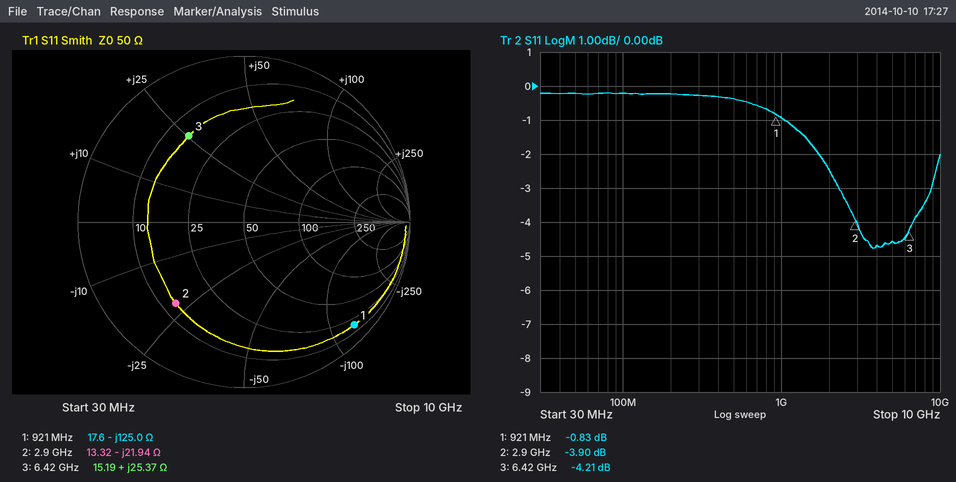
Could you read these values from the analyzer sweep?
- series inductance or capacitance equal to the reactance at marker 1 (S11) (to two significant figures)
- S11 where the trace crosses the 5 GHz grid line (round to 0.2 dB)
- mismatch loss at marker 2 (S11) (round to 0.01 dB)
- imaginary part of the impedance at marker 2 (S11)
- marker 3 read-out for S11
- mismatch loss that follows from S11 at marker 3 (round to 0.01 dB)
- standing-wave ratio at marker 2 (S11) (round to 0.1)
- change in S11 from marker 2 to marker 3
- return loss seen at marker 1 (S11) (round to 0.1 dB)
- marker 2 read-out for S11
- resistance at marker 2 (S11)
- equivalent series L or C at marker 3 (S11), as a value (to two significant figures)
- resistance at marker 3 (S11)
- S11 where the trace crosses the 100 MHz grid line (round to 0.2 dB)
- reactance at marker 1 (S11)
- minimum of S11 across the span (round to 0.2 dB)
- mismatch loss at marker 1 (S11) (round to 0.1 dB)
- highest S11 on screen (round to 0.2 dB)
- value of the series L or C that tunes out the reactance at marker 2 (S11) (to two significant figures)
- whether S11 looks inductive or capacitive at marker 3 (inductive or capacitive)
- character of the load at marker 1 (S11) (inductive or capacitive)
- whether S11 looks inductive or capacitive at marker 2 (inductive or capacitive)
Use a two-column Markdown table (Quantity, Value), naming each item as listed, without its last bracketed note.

| Quantity | Value |
|---|---|
| series inductance or capacitance equal to the reactance at marker 1 (S11) | 1.4 pF |
| S11 where the trace crosses the 5 GHz grid line | -4.6 dB |
| mismatch loss at marker 2 (S11) | 2.27 dB |
| imaginary part of the impedance at marker 2 | -21.94 Ω |
| marker 3 read-out for S11 | -4.21 dB |
| mismatch loss that follows from S11 at marker 3 | 2.07 dB |
| standing-wave ratio at marker 2 (S11) | 4.5 |
| change in S11 from marker 2 to marker 3 | -0.31 dB |
| return loss seen at marker 1 (S11) | 0.8 dB |
| marker 2 read-out for S11 | -3.90 dB |
| resistance at marker 2 | 13.32 Ω |
| equivalent series L or C at marker 3 (S11), as a value | 630 pH |
| resistance at marker 3 | 15.19 Ω |
| S11 where the trace crosses the 100 MHz grid line | -0.2 dB |
| reactance at marker 1 | -125.0 Ω |
| minimum of S11 across the span | -4.8 dB |
| mismatch loss at marker 1 (S11) | 7.6 dB |
| highest S11 on screen | -0.2 dB |
| value of the series L or C that tunes out the reactance at marker 2 (S11) | 1.2 nH |
| whether S11 looks inductive or capacitive at marker 3 | inductive |
| character of the load at marker 1 (S11) | capacitive |
| whether S11 looks inductive or capacitive at marker 2 | capacitive |
